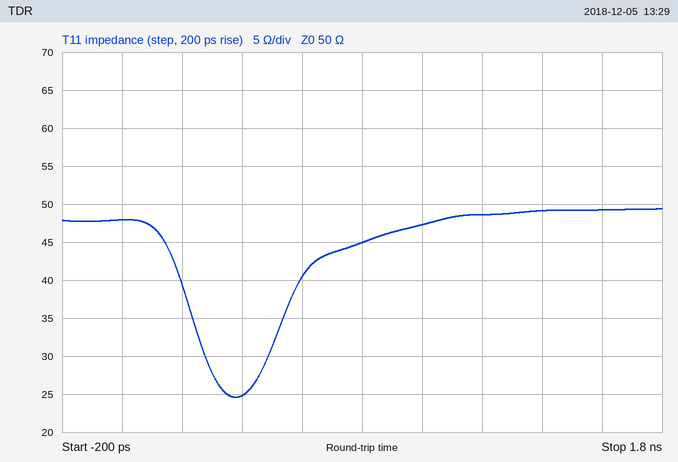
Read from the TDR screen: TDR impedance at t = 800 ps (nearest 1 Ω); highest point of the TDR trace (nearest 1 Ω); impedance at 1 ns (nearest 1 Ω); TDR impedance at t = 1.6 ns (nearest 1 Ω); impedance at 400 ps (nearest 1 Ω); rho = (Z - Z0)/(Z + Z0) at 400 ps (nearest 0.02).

45 Ω
49 Ω
47 Ω
49 Ω
25 Ω
-0.34
